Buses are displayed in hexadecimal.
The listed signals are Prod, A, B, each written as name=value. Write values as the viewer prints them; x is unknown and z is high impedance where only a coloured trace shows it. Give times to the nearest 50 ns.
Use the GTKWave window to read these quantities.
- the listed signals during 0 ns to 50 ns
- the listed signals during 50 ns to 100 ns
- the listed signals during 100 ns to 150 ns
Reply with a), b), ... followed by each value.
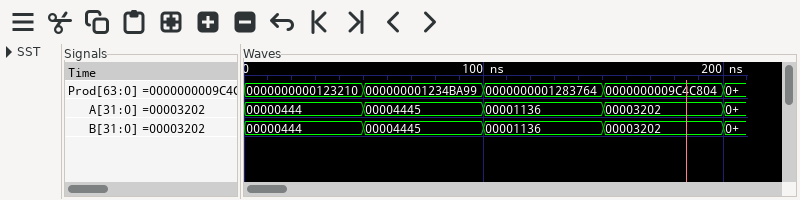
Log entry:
a) Prod=0000000000123210, A=00000444, B=00000444
b) Prod=000000001234BA99, A=00004445, B=00004445
c) Prod=0000000001283764, A=00001136, B=00001136
